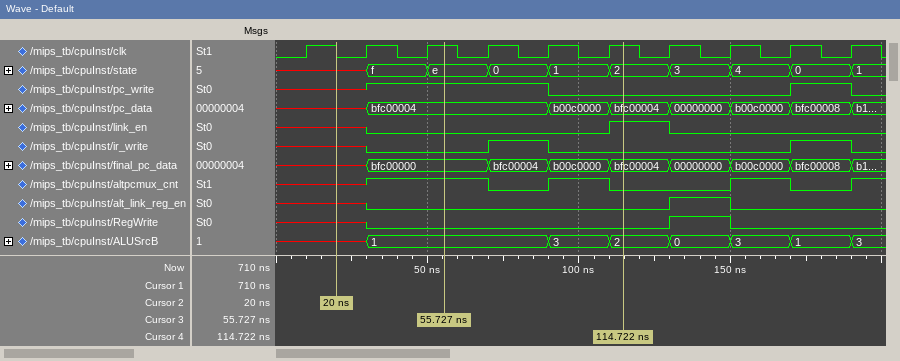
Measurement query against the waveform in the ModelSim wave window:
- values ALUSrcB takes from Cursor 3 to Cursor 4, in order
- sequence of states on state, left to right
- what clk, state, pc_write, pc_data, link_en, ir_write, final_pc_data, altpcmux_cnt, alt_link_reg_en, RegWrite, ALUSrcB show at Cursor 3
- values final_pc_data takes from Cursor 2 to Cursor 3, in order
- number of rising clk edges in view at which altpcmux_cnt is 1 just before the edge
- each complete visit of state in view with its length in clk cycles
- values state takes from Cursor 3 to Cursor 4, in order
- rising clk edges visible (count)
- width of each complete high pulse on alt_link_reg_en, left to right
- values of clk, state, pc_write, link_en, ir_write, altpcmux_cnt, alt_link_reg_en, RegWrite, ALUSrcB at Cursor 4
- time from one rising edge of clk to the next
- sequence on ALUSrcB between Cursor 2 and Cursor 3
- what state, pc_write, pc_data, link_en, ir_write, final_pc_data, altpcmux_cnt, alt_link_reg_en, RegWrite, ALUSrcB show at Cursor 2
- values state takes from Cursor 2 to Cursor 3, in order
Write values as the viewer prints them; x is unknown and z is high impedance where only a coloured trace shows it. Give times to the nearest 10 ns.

1, 3, 2
x, f, e, 0, 1, 2, 3, 4, 0, 1
clk=1, state=e, pc_write=1, pc_data=bfc00004, link_en=0, ir_write=0, final_pc_data=bfc00000, altpcmux_cnt=1, alt_link_reg_en=0, RegWrite=0, ALUSrcB=1
x, bfc00000
4
f: 1, e: 1, 0: 1, 1: 1, 2: 1, 3: 1, 4: 1, 0: 1
e, 0, 1, 2
10
20 ns
clk=1, state=2, pc_write=0, link_en=1, ir_write=0, altpcmux_cnt=0, alt_link_reg_en=0, RegWrite=0, ALUSrcB=2
20 ns
x, 1
state=x, pc_write=x, pc_data=x, link_en=x, ir_write=x, final_pc_data=x, altpcmux_cnt=x, alt_link_reg_en=x, RegWrite=x, ALUSrcB=x
x, f, e
